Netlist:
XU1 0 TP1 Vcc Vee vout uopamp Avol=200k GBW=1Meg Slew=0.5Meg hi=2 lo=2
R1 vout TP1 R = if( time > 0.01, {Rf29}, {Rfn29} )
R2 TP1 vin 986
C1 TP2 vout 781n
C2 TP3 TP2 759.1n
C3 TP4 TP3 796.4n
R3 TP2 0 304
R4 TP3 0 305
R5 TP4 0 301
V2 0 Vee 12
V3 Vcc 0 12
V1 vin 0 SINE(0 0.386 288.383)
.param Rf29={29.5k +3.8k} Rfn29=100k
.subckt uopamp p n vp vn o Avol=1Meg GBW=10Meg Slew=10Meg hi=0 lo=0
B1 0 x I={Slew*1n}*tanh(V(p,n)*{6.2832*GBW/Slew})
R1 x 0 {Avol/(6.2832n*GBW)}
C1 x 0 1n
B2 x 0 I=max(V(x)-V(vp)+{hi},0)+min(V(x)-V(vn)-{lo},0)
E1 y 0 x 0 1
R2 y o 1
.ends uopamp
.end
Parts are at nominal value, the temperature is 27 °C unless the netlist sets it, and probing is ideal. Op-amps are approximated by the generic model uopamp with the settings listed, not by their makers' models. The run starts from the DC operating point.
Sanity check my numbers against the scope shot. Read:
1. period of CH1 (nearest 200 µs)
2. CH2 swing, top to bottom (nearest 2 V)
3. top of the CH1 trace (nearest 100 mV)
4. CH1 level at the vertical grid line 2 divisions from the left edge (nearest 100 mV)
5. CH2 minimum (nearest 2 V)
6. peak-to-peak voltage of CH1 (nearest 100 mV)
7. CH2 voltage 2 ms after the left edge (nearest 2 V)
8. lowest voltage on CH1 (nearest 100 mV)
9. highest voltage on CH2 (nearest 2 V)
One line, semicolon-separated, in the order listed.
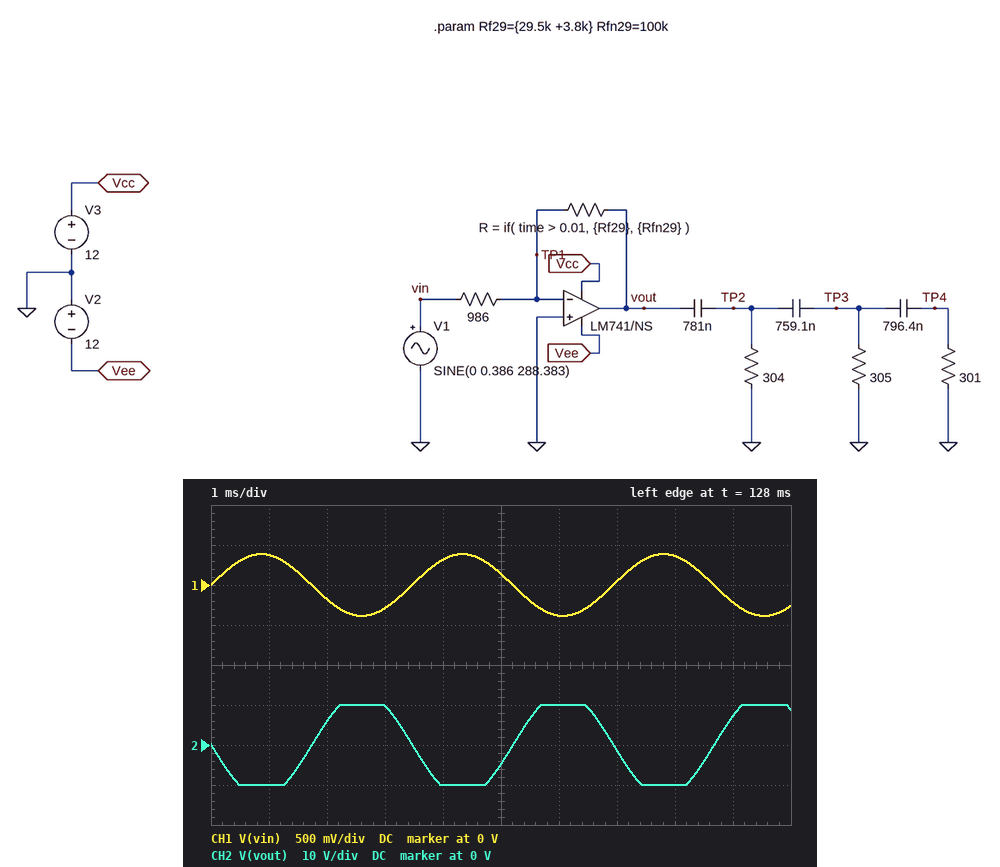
3.4 ms; 20 V; 400 mV; -200 mV; -10 V; 800 mV; 6 V; -400 mV; 10 V
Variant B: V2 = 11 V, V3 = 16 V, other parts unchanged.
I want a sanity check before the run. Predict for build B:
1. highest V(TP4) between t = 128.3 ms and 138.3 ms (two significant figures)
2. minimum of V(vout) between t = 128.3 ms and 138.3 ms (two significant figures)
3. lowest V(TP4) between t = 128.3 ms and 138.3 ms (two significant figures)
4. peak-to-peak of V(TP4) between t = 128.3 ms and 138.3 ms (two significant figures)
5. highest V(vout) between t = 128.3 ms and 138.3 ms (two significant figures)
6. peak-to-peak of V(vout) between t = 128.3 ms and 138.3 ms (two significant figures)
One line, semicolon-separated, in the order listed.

850 mV; -9.0 V; -500 mV; 1.3 V; 13 V; 22 V
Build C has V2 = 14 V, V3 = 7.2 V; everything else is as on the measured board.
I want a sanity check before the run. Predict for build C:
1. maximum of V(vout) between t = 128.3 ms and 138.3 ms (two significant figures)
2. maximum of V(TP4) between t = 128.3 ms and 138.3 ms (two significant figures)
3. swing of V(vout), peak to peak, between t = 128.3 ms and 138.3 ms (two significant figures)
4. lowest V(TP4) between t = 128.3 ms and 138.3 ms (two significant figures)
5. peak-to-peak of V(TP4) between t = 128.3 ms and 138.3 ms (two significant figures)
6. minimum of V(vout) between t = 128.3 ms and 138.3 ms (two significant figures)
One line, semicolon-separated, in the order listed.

5.2 V; 670 mV; 17 V; -870 mV; 1.5 V; -12 V
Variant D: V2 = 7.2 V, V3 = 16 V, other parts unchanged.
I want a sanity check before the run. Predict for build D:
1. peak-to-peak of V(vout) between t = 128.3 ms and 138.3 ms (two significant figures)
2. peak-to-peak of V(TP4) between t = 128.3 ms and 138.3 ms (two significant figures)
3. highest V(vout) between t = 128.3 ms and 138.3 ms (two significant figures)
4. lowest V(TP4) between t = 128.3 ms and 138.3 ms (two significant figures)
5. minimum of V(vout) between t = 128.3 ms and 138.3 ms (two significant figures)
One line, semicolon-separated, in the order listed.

18 V; 1.4 V; 13 V; -500 mV; -5.2 V
